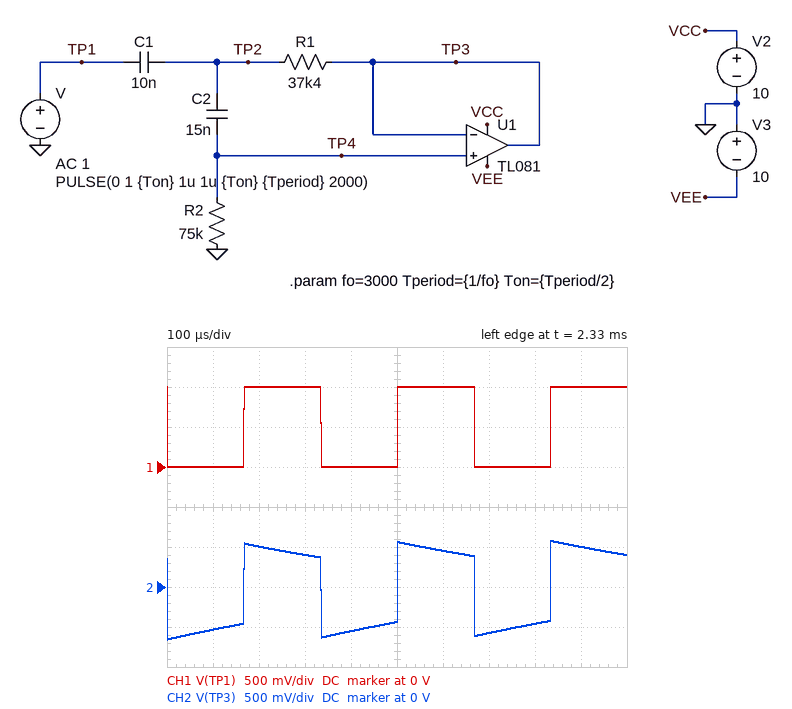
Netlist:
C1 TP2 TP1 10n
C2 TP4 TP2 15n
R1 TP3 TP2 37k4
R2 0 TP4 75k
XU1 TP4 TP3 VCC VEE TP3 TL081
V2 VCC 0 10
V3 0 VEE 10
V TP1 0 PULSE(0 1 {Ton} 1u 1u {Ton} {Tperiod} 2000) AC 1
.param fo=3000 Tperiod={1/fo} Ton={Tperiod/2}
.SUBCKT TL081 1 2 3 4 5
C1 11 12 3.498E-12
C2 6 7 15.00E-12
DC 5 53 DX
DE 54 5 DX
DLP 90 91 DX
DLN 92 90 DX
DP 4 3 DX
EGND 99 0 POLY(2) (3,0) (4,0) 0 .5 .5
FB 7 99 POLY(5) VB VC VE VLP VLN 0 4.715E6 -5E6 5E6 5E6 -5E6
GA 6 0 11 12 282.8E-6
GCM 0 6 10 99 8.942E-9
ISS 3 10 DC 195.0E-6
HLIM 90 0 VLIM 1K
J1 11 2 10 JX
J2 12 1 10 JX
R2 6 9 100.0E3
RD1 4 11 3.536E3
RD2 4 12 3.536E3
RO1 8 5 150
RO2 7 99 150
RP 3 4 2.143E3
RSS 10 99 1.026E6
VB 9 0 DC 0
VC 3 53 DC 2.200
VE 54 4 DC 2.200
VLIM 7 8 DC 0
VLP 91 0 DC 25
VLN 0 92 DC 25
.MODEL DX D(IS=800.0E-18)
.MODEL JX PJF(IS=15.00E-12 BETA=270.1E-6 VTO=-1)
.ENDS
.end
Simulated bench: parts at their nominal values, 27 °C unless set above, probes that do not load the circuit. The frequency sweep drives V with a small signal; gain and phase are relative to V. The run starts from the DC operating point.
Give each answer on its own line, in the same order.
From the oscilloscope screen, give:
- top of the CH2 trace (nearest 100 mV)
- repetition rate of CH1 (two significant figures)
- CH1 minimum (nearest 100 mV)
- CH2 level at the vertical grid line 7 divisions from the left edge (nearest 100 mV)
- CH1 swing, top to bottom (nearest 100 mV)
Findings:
600 mV
3.0 kHz
0 V
-600 mV
1.0 V
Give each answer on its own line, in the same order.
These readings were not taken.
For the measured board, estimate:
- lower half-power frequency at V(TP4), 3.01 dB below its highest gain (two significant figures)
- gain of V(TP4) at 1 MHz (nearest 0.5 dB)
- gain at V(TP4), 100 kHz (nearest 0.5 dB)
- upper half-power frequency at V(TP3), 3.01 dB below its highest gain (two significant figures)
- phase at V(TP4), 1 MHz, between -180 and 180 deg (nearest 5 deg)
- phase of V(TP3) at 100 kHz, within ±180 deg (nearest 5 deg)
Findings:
250 Hz
0 dB
0 dB
4.8 MHz
0 deg
0 deg
